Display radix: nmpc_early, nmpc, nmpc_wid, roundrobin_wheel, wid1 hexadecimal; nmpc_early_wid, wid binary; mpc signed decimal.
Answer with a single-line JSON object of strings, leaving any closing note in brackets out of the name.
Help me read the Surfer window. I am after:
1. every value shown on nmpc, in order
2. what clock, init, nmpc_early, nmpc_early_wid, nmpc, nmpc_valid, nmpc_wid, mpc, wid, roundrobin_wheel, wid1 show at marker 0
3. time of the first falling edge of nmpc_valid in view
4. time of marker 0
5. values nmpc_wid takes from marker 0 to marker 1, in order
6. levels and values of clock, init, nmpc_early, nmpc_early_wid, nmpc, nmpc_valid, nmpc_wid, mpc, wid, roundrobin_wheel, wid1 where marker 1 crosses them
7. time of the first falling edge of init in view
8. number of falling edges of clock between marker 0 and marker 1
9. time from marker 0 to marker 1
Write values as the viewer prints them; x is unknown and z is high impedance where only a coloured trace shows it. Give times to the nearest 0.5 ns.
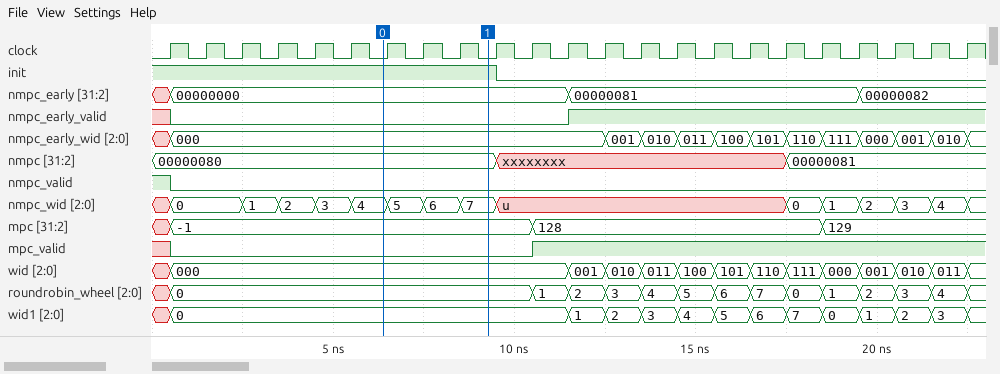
{"every value shown on nmpc, in order": "00000080, xxxxxxxx, 00000081", "what clock, init, nmpc_early, nmpc_early_wid, nmpc, nmpc_valid, nmpc_wid, mpc, wid, roundrobin_wheel, wid1 show at marker 0": "clock=0, init=1, nmpc_early=00000000, nmpc_early_wid=000, nmpc=00000080, nmpc_valid=0, nmpc_wid=4, mpc=-1, wid=000, roundrobin_wheel=0, wid1=0", "time of the first falling edge of nmpc_valid in view": "0.5 ns", "time of marker 0": "6.5 ns", "values nmpc_wid takes from marker 0 to marker 1, in order": "4, 5, 6, 7", "levels and values of clock, init, nmpc_early, nmpc_early_wid, nmpc, nmpc_valid, nmpc_wid, mpc, wid, roundrobin_wheel, wid1 where marker 1 crosses them": "clock=0, init=1, nmpc_early=00000000, nmpc_early_wid=000, nmpc=00000080, nmpc_valid=0, nmpc_wid=7, mpc=-1, wid=000, roundrobin_wheel=0, wid1=0", "time of the first falling edge of init in view": "9.5 ns", "number of falling edges of clock between marker 0 and marker 1": "3", "time from marker 0 to marker 1": "3 ns"}
